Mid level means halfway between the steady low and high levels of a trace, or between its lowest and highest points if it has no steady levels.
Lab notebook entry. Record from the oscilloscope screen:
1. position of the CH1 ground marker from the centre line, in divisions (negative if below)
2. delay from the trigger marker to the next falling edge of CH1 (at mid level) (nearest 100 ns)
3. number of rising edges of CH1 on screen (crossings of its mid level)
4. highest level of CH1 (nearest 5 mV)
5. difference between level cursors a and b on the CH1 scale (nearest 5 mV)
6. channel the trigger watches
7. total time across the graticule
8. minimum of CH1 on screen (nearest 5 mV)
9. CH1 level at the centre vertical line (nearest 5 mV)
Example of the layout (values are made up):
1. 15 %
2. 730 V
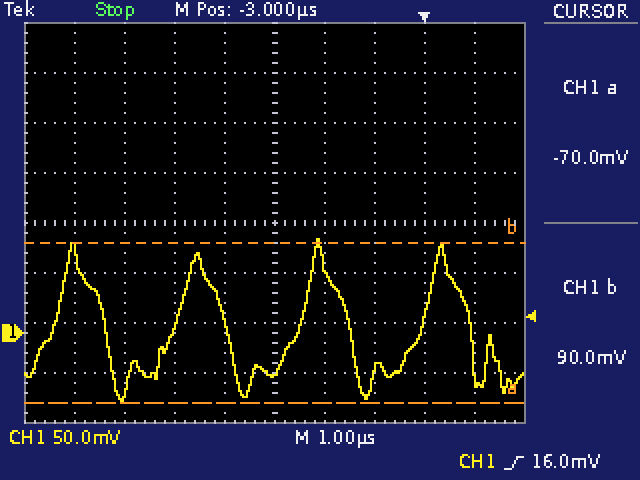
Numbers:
1. -2.2 div
2. 900 ns
3. 4
4. 95 mV
5. 160 mV
6. CH1
7. 10 µs
8. -70 mV
9. -40 mV
